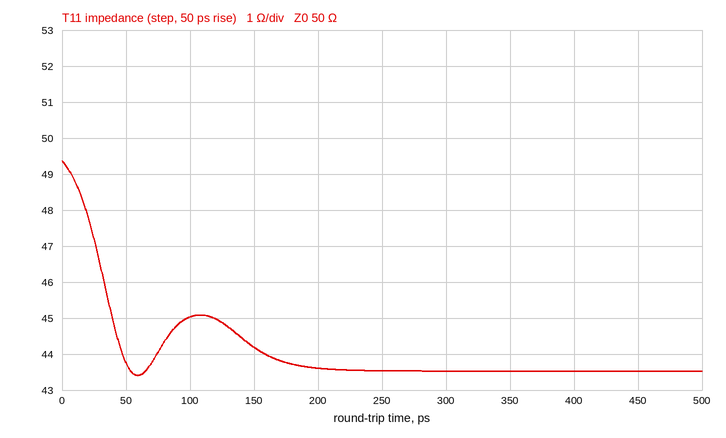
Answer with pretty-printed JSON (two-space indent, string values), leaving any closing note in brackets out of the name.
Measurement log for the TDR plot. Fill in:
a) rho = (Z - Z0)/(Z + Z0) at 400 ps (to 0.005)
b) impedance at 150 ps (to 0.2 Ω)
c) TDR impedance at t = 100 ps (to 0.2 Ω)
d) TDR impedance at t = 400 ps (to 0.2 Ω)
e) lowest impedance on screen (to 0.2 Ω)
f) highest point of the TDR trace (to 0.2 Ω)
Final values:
{
  "rho = (Z - Z0)/(Z + Z0) at 400 ps": "-0.070",
  "impedance at 150 ps": "44.2 Ω",
  "TDR impedance at t = 100 ps": "45.0 Ω",
  "TDR impedance at t = 400 ps": "43.6 Ω",
  "lowest impedance on screen": "43.4 Ω",
  "highest point of the TDR trace": "49.4 Ω"
}
